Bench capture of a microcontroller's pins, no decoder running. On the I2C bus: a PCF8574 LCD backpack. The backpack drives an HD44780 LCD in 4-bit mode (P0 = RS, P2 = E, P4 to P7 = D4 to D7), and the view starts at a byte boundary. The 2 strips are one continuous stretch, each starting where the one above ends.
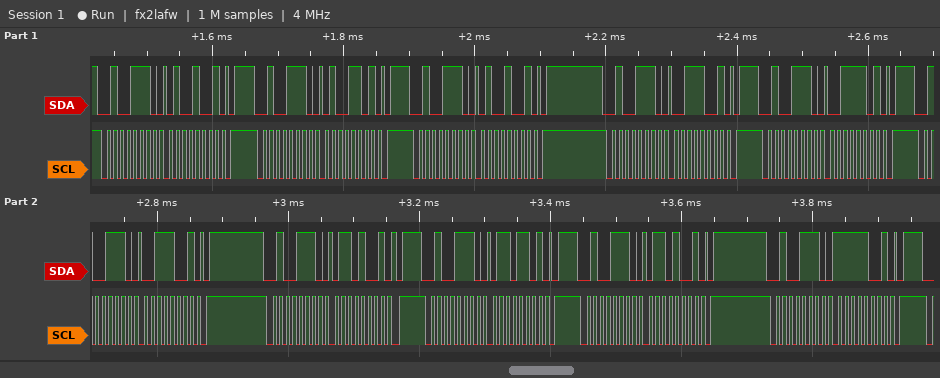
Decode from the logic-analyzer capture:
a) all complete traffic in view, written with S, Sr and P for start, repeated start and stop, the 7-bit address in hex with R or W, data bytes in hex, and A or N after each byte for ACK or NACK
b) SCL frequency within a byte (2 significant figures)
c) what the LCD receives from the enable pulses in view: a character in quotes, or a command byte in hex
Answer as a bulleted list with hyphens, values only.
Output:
- S 27W A 49 A P S 27W A 4D A P S 27W A 49 A P S 27W A 39 A P S 27W A 3D A P S 27W A 39 A P S 27W A 69 A P S 27W A 6D A P S 27W A 69 A P S 27W A F9 A P
- 100 kHz
- 'C'
